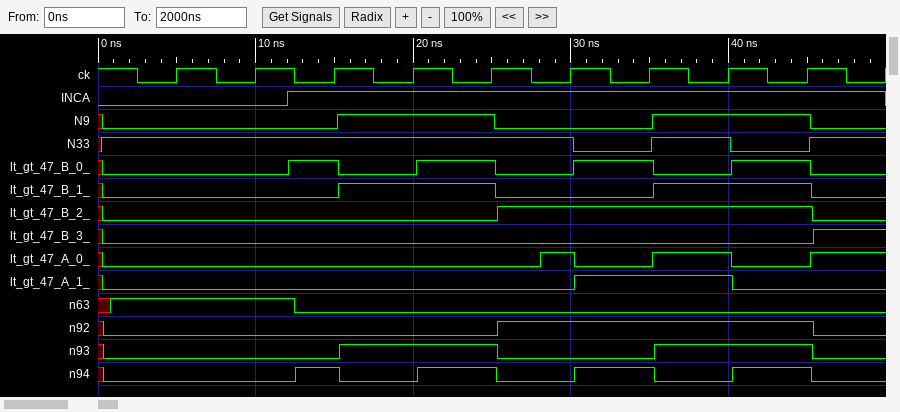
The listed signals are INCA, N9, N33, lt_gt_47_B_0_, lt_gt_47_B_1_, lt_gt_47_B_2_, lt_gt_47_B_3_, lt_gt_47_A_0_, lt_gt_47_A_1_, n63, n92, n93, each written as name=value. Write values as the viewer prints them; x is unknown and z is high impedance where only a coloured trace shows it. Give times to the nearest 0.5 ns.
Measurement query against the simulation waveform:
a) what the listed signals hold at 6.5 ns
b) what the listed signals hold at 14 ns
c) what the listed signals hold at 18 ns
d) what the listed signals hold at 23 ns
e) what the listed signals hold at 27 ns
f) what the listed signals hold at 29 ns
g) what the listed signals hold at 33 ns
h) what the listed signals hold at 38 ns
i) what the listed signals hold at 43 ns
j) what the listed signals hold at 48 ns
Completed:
INCA=0, N9=0, N33=1, lt_gt_47_B_0_=0, lt_gt_47_B_1_=0, lt_gt_47_B_2_=0, lt_gt_47_B_3_=0, lt_gt_47_A_0_=0, lt_gt_47_A_1_=0, n63=1, n92=0, n93=0
INCA=1, N9=0, N33=1, lt_gt_47_B_0_=1, lt_gt_47_B_1_=0, lt_gt_47_B_2_=0, lt_gt_47_B_3_=0, lt_gt_47_A_0_=0, lt_gt_47_A_1_=0, n63=0, n92=0, n93=0
INCA=1, N9=1, N33=1, lt_gt_47_B_0_=0, lt_gt_47_B_1_=1, lt_gt_47_B_2_=0, lt_gt_47_B_3_=0, lt_gt_47_A_0_=0, lt_gt_47_A_1_=0, n63=0, n92=0, n93=1
INCA=1, N9=1, N33=1, lt_gt_47_B_0_=1, lt_gt_47_B_1_=1, lt_gt_47_B_2_=0, lt_gt_47_B_3_=0, lt_gt_47_A_0_=0, lt_gt_47_A_1_=0, n63=0, n92=0, n93=1
INCA=1, N9=0, N33=1, lt_gt_47_B_0_=0, lt_gt_47_B_1_=0, lt_gt_47_B_2_=1, lt_gt_47_B_3_=0, lt_gt_47_A_0_=0, lt_gt_47_A_1_=0, n63=0, n92=1, n93=0
INCA=1, N9=0, N33=1, lt_gt_47_B_0_=0, lt_gt_47_B_1_=0, lt_gt_47_B_2_=1, lt_gt_47_B_3_=0, lt_gt_47_A_0_=1, lt_gt_47_A_1_=0, n63=0, n92=1, n93=0
INCA=1, N9=0, N33=0, lt_gt_47_B_0_=1, lt_gt_47_B_1_=0, lt_gt_47_B_2_=1, lt_gt_47_B_3_=0, lt_gt_47_A_0_=0, lt_gt_47_A_1_=1, n63=0, n92=1, n93=0
INCA=1, N9=1, N33=1, lt_gt_47_B_0_=0, lt_gt_47_B_1_=1, lt_gt_47_B_2_=1, lt_gt_47_B_3_=0, lt_gt_47_A_0_=1, lt_gt_47_A_1_=1, n63=0, n92=1, n93=1
INCA=1, N9=1, N33=0, lt_gt_47_B_0_=1, lt_gt_47_B_1_=1, lt_gt_47_B_2_=1, lt_gt_47_B_3_=0, lt_gt_47_A_0_=0, lt_gt_47_A_1_=0, n63=0, n92=1, n93=1
INCA=1, N9=0, N33=1, lt_gt_47_B_0_=0, lt_gt_47_B_1_=0, lt_gt_47_B_2_=0, lt_gt_47_B_3_=1, lt_gt_47_A_0_=1, lt_gt_47_A_1_=0, n63=0, n92=0, n93=0
